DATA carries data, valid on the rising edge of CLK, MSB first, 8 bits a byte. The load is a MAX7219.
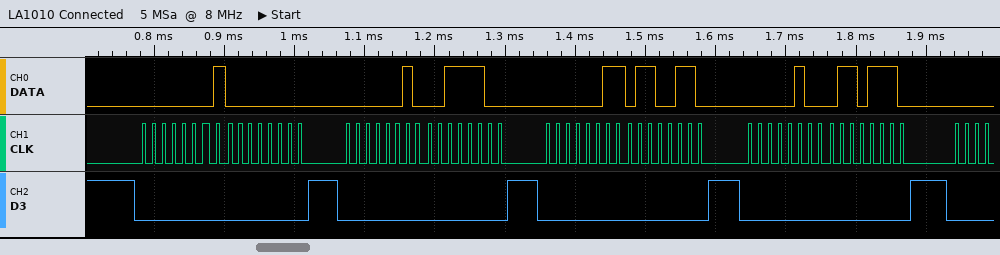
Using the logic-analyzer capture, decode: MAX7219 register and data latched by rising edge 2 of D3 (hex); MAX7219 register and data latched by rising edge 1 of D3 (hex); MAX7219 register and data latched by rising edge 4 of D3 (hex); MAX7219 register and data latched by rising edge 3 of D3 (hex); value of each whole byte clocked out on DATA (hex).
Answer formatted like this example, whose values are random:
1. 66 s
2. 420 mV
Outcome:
1. register 0x2, data 0x3C
2. register 0x1, data 0x00
3. register 0x4, data 0x6E
4. register 0x3, data 0x66
5. 01 00 02 3C 03 66 04 6E
